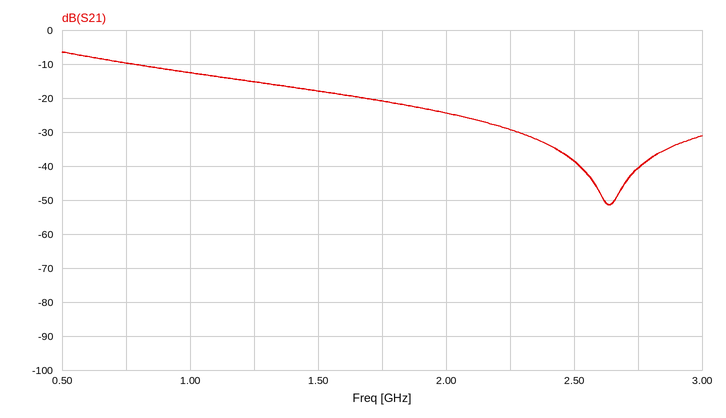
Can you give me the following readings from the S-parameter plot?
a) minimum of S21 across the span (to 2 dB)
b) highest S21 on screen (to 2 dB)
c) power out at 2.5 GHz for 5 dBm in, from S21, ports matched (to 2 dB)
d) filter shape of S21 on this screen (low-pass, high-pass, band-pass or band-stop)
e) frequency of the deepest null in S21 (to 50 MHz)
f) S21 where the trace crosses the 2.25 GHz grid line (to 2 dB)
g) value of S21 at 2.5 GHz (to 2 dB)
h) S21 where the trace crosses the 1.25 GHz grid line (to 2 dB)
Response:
-52 dB
-6 dB
-34 dBm
low-pass
2.65 GHz
-30 dB
-38 dB
-16 dB
